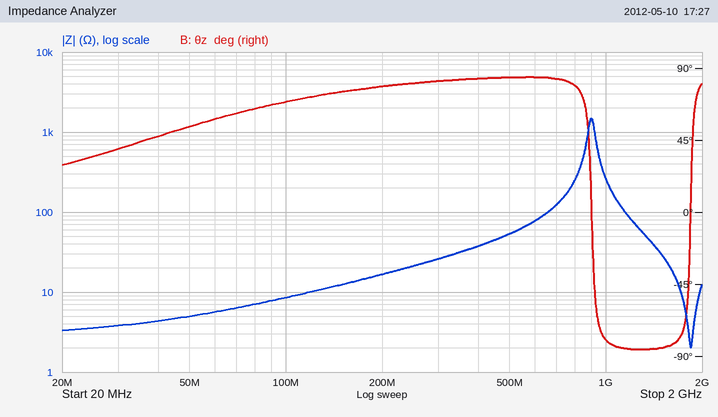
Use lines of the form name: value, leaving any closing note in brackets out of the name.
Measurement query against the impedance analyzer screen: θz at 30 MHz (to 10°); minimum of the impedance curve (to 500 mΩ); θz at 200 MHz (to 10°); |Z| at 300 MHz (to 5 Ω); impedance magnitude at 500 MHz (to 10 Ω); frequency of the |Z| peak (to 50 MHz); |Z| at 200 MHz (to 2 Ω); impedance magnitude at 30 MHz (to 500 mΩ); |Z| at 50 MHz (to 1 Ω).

θz at 30 MHz: 40°
minimum of the impedance curve: 2.0 Ω
θz at 200 MHz: 80°
|Z| at 300 MHz: 25 Ω
impedance magnitude at 500 MHz: 50 Ω
frequency of the |Z| peak: 900 MHz
|Z| at 200 MHz: 16 Ω
impedance magnitude at 30 MHz: 4.0 Ω
|Z| at 50 MHz: 5 Ω
